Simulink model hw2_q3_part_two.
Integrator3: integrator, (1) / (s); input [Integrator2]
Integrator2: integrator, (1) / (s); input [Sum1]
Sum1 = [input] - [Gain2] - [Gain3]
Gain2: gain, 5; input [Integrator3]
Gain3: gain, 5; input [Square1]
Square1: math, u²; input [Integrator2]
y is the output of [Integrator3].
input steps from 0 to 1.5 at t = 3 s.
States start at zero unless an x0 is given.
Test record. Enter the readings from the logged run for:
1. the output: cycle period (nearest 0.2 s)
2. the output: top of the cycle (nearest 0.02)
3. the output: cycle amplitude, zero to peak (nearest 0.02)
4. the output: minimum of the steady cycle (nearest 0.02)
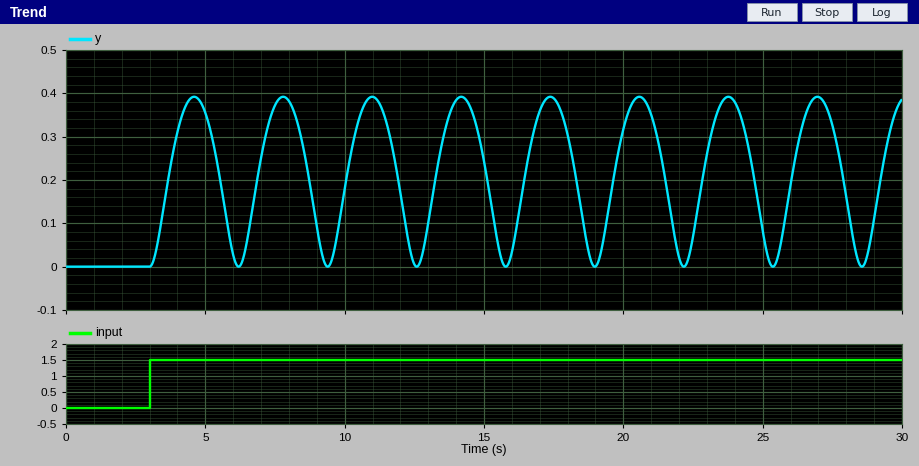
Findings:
3.2 s
0.40
0.20
0.00
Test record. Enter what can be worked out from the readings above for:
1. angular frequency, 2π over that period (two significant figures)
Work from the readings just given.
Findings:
2.0 rad/s
